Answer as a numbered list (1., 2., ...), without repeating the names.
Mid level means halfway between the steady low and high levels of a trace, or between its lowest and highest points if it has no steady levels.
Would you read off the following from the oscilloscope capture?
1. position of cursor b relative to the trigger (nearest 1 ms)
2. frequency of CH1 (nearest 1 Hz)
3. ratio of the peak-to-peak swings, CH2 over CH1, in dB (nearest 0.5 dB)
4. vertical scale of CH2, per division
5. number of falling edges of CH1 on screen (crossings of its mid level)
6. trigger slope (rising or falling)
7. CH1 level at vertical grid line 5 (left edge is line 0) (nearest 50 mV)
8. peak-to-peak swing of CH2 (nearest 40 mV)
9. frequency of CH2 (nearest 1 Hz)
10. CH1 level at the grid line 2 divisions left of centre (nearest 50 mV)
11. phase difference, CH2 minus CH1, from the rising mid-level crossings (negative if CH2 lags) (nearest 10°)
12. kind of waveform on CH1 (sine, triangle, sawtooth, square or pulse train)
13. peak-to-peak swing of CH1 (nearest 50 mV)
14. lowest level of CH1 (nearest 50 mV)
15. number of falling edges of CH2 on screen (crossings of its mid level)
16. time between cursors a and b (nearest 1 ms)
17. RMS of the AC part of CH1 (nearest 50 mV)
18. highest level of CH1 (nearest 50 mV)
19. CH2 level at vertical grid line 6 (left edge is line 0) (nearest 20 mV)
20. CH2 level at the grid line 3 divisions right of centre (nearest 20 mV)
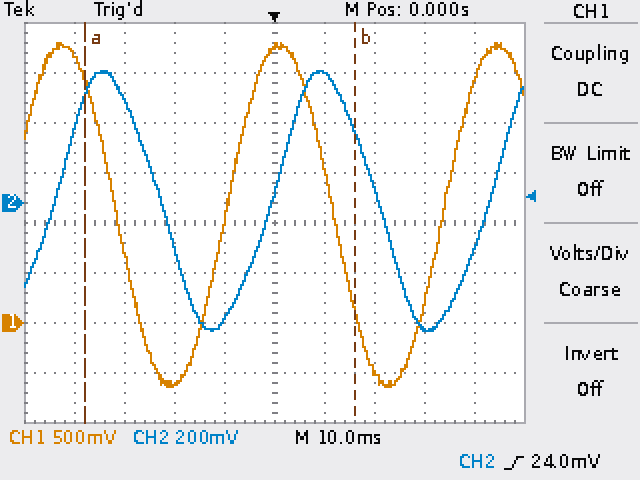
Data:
1. +16 ms
2. 23 Hz
3. -10.5 dB
4. 200 mV
5. 2
6. rising
7. 2.75 V
8. 1.04 V
9. 23 Hz
10. -600 mV
11. -80°
12. sine
13. 3.45 V
14. -650 mV
15. 2
16. 54 ms
17. 1.20 V
18. 2.80 V
19. 520 mV
20. -500 mV
